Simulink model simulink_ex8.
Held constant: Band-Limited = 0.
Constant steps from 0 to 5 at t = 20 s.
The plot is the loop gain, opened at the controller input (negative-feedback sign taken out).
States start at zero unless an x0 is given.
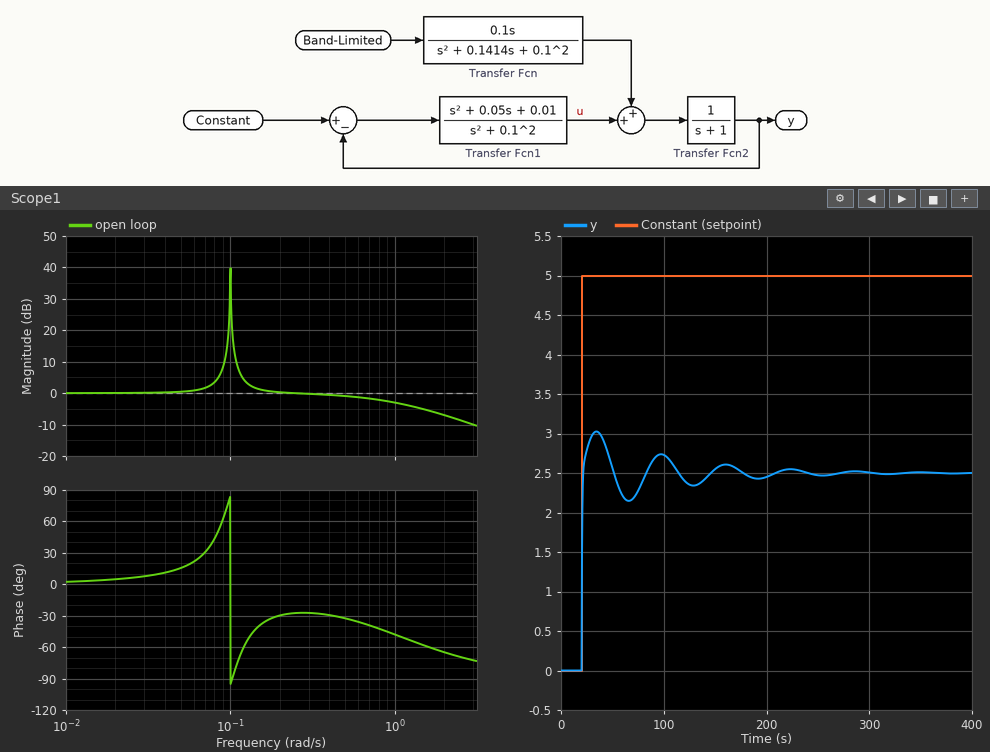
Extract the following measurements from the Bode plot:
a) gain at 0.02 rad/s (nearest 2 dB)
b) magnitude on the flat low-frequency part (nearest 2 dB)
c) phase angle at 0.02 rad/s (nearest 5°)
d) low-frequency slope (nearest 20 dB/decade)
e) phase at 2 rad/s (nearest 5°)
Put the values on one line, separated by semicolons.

0 dB; 0 dB; 5°; 0 dB/decade; -65°
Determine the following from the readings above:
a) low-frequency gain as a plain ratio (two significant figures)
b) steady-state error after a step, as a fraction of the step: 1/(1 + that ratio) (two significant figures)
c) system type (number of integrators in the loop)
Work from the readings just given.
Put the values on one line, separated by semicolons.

1.0; 0.50; 0
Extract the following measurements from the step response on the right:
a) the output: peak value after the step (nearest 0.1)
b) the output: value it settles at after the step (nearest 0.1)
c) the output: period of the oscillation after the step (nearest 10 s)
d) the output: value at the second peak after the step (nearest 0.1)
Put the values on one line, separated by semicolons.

3.0; 2.5; 60 s; 2.7
